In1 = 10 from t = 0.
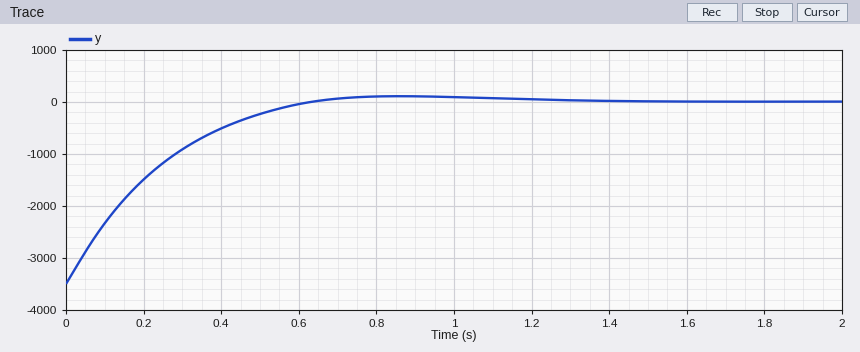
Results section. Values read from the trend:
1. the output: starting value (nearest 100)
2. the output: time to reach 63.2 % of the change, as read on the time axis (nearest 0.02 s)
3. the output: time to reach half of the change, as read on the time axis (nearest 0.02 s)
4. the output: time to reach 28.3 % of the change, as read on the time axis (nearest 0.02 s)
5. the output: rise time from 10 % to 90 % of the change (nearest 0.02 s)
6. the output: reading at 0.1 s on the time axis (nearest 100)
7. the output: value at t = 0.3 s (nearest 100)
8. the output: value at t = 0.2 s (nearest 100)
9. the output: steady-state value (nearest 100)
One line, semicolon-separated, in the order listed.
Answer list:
-3500; 0.24 s; 0.16 s; 0.08 s; 0.42 s; -2300; -900; -1500; 0
